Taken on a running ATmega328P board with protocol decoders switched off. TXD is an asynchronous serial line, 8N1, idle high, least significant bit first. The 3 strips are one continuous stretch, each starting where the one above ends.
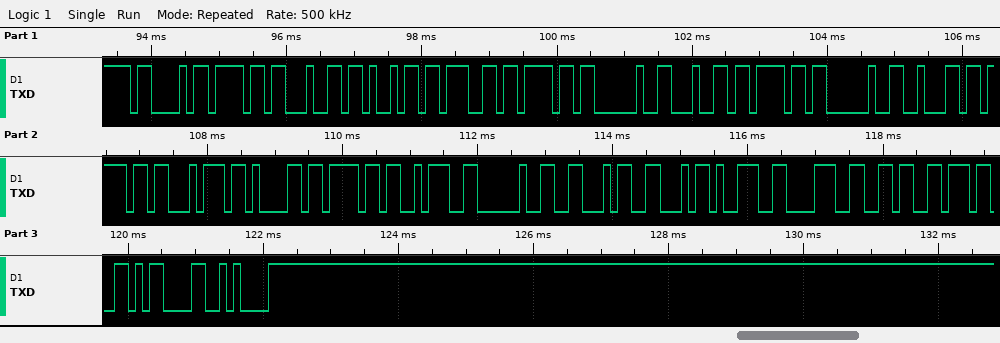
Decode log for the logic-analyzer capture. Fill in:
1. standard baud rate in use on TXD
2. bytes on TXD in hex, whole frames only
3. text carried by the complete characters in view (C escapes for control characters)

9600 baud
43 6F 64 69 67 6F 20 64 6F 20 62 6F 74 61 6F 3A 20 46 46 39 38 36 37 0D 0A
"Codigo do botao: FF9867\r\n"
